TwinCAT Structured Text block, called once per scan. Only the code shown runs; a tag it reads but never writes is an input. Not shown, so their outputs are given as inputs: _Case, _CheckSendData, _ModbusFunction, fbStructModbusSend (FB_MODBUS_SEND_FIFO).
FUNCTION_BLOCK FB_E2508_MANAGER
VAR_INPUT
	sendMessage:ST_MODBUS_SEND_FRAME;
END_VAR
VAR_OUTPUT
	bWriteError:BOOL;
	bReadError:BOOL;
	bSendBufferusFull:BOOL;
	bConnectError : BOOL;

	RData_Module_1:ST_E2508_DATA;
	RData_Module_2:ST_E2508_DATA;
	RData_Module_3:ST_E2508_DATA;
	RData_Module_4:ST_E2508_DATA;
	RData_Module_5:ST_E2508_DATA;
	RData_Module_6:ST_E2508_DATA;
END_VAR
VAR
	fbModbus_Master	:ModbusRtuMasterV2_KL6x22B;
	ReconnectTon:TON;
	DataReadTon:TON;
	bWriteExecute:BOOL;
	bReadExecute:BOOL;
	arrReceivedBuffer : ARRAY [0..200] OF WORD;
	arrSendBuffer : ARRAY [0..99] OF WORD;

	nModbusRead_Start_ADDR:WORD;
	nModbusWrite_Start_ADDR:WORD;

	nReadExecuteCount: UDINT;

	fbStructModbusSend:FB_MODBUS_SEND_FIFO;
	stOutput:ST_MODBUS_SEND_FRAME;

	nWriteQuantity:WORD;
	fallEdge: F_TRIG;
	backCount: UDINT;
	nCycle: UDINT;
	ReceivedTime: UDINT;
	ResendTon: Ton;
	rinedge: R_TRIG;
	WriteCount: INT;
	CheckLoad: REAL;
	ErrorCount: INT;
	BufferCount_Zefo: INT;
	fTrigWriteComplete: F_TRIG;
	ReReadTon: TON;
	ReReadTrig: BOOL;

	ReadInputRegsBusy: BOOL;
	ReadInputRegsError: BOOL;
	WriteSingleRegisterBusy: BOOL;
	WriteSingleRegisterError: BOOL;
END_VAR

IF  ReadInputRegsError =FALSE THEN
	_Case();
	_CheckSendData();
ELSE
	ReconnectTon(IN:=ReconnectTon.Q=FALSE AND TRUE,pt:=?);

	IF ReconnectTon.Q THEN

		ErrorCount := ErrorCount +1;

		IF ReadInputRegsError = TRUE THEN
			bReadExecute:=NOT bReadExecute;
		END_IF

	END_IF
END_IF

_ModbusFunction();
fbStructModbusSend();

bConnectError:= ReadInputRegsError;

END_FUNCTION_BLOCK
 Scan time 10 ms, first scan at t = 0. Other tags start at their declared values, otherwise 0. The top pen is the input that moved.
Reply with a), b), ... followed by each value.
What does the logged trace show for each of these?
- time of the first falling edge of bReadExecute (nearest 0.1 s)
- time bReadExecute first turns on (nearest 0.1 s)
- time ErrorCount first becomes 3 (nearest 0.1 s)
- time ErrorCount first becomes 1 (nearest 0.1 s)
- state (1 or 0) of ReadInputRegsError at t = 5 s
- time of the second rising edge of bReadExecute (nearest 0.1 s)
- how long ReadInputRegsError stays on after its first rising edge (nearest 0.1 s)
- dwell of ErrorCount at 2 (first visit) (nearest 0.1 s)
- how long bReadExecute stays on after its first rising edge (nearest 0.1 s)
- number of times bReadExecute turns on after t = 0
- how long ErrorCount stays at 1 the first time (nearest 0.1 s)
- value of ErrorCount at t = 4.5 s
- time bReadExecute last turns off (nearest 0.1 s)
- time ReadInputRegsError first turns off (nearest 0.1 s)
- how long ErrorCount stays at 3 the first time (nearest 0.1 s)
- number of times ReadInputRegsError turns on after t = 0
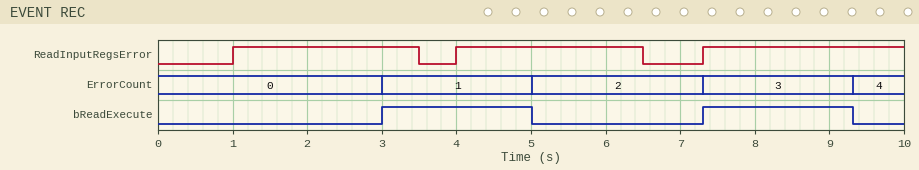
a) 5.0 s
b) 3.0 s
c) 7.3 s
d) 3.0 s
e) 1
f) 7.3 s
g) 2.5 s
h) 2.3 s
i) 2.0 s
j) 2
k) 2.0 s
l) 1
m) 9.3 s
n) 3.5 s
o) 2.0 s
p) 3
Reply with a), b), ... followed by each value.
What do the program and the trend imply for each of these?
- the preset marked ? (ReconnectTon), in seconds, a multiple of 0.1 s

a) 2.0 s
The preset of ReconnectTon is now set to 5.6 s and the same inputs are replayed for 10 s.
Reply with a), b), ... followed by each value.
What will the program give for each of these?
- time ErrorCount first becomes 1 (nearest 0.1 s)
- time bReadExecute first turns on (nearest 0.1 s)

a) 7.3 s
b) 7.3 s
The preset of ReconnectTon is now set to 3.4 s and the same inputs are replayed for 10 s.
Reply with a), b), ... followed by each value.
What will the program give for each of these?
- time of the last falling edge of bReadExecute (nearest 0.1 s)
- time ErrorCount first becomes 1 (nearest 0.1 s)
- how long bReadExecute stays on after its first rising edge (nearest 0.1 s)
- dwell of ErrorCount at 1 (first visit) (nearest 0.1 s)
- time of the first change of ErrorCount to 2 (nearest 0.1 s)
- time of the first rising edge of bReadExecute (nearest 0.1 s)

a) 7.8 s
b) 4.4 s
c) 3.4 s
d) 3.4 s
e) 7.8 s
f) 4.4 s
